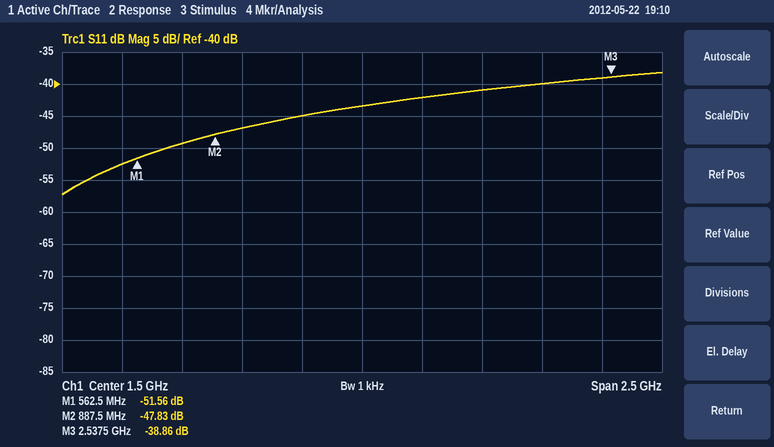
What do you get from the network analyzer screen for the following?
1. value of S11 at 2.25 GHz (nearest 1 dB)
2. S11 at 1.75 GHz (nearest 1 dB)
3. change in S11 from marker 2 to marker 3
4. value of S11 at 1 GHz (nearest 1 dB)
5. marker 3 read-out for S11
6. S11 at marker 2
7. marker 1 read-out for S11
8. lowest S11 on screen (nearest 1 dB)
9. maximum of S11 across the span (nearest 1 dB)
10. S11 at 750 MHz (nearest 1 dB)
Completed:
-40 dB
-42 dB
8.97 dB
-47 dB
-38.86 dB
-47.83 dB
-51.56 dB
-57 dB
-38 dB
-49 dB
